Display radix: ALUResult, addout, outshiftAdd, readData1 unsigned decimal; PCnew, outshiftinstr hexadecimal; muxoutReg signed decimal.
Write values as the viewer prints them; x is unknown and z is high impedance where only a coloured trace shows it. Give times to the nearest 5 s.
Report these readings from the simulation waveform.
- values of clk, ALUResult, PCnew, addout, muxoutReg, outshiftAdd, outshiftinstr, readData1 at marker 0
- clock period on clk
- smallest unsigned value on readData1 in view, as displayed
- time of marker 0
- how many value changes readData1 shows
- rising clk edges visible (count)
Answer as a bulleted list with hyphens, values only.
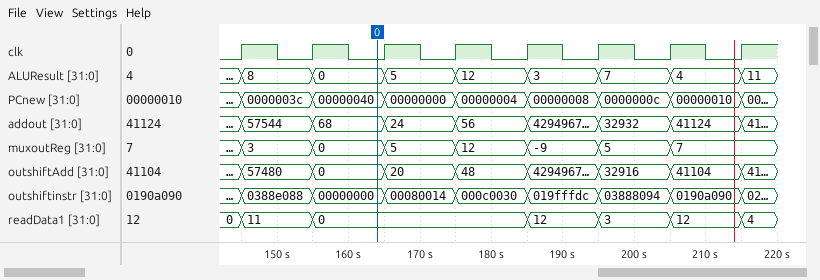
- clk=0, ALUResult=0, PCnew=00000040, addout=68, muxoutReg=0, outshiftAdd=0, outshiftinstr=00000000, readData1=0
- 10 s
- 0
- 165 s
- 6
- 8
